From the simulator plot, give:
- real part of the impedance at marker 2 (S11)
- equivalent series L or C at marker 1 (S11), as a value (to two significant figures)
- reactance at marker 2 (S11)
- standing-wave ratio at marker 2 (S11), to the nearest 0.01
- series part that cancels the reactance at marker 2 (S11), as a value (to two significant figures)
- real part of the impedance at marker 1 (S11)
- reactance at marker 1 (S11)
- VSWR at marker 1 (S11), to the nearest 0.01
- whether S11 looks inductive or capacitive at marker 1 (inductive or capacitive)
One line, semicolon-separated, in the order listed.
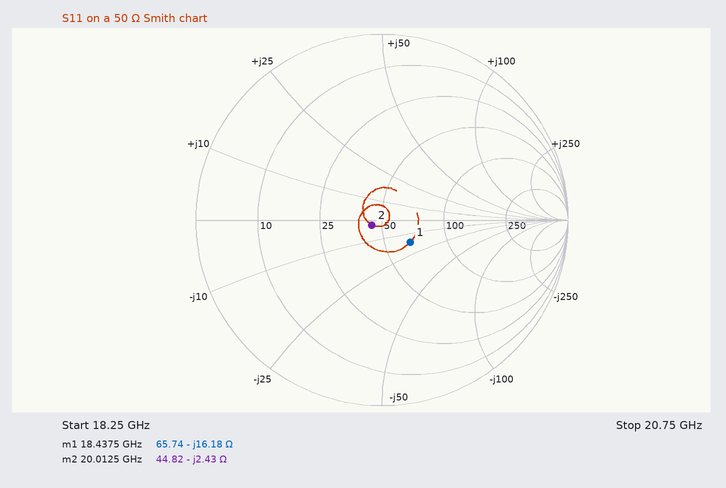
44.82 Ω; 530 fF; -2.43 Ω; 1.13; 19 pH; 65.74 Ω; -16.18 Ω; 1.48; capacitive
